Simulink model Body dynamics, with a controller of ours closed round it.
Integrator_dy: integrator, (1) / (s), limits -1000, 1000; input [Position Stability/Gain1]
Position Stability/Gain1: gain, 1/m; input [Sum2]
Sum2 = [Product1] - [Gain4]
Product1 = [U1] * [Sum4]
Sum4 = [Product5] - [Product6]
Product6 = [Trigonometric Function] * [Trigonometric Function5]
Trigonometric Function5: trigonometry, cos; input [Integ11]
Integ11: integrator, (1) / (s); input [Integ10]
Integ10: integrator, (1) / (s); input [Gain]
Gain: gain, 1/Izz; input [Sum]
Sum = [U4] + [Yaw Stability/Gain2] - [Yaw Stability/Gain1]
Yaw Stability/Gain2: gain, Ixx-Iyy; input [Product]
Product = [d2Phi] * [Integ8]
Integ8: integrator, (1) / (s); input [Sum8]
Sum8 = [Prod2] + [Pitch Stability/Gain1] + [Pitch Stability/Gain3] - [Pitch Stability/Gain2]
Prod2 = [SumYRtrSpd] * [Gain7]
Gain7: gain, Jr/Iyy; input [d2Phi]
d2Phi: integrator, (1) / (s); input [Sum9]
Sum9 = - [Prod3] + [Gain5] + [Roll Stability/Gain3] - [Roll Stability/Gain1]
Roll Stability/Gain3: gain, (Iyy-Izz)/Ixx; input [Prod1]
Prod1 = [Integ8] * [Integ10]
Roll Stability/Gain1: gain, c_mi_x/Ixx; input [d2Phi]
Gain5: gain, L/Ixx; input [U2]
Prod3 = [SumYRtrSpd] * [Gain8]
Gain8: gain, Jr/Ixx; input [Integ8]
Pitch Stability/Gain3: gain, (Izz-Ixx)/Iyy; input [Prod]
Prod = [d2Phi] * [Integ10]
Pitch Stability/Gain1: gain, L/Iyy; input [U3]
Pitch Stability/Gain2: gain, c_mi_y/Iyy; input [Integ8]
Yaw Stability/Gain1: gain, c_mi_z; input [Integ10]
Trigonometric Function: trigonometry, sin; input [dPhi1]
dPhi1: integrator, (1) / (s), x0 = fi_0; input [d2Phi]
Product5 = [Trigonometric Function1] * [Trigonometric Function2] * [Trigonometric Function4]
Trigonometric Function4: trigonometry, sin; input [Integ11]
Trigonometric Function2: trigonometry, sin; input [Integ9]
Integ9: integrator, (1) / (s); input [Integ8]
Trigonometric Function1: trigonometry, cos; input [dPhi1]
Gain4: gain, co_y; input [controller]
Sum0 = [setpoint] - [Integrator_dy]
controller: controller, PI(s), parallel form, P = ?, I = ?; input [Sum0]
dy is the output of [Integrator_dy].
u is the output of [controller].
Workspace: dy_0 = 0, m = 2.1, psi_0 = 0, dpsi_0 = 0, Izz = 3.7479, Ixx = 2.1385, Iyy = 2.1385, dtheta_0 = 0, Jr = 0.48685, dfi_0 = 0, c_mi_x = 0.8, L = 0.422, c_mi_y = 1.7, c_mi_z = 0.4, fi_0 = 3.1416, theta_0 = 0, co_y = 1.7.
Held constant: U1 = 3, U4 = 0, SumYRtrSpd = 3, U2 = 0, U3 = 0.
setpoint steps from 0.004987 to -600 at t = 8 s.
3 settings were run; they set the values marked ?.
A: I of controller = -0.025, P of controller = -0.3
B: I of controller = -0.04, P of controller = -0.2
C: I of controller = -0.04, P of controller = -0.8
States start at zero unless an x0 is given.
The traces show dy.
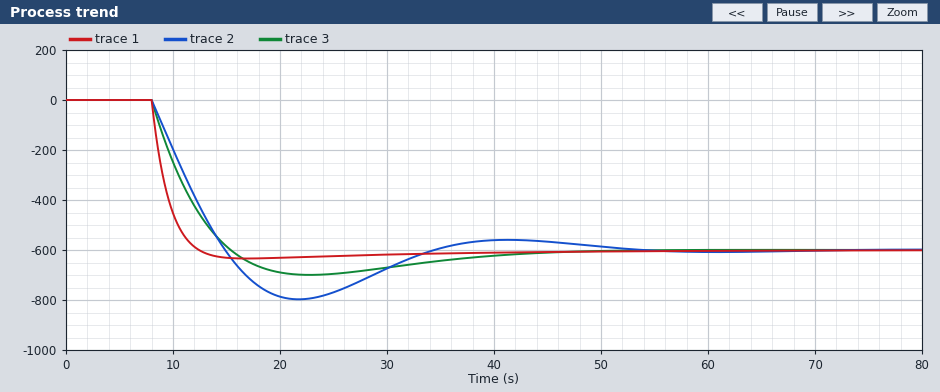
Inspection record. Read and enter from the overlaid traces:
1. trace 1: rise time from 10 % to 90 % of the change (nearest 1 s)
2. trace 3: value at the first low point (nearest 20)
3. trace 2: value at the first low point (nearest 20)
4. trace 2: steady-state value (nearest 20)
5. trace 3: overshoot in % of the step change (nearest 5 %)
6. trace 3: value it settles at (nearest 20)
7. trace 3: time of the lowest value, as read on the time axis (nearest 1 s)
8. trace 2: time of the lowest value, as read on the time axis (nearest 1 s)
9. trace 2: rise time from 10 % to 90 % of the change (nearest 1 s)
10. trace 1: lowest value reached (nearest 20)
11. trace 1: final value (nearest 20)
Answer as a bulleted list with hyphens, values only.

- 3 s
- -700
- -800
- -600
- 15 %
- -600
- 23 s
- 22 s
- 5 s
- -640
- -600
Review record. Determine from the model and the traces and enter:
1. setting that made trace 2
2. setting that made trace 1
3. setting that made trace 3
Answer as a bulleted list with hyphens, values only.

- B
- C
- A
